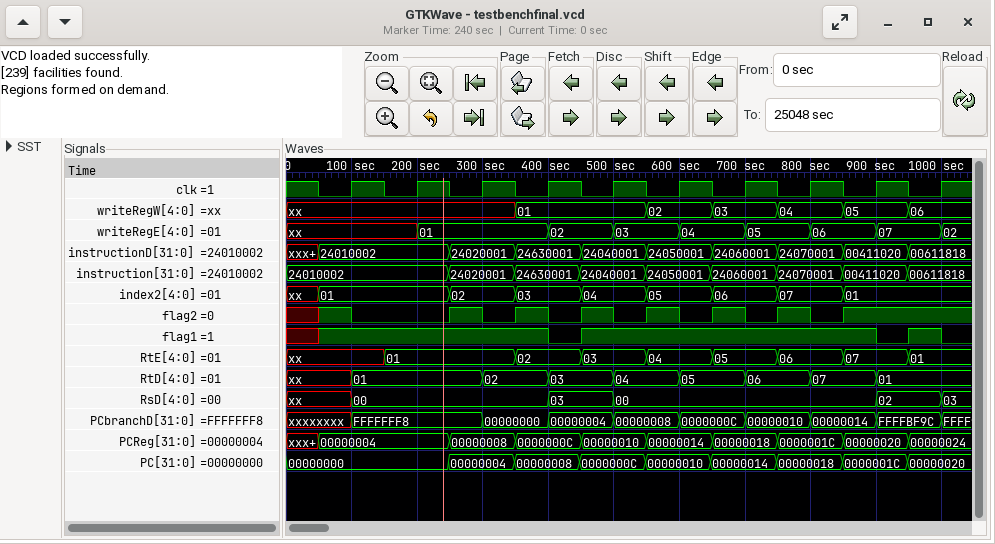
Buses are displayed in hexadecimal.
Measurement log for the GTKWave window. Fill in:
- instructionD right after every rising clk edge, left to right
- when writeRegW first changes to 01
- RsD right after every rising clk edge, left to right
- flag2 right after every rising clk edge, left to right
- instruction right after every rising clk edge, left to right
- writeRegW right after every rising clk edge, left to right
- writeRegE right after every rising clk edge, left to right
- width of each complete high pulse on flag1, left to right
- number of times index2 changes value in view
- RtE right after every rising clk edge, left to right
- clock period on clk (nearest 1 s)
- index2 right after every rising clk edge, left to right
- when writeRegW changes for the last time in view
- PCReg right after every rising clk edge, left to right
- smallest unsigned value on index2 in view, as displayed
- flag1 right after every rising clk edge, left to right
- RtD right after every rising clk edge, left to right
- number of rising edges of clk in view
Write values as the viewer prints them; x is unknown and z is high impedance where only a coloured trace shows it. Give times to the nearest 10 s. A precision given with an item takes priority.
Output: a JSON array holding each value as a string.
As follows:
["24010002, 24010002, 24020001, 24630001, 24040001, 24050001, 24060001, 24070001, 00411020, 00611818", "350 s", "00, 00, 00, 03, 00, 00, 00, 00, 02, 03", "0 0 0 0 0 0 0 0 1 1", "24010002, 24010002, 24020001, 24630001, 24040001, 24050001, 24060001, 24070001, 00411020, 00611818", "xx, xx, xx, 01, 01, 02, 03, 04, 05, 06", "xx, 01, 01, 02, 03, 04, 05, 06, 07, 02", "450 s, 50 s", "8", "xx, 01, 01, 02, 03, 04, 05, 06, 07, 01", "100 s", "01, 01, 02, 03, 04, 05, 06, 07, 01, 01", "950 s", "00000004, 00000004, 00000008, 0000000C, 00000010, 00000014, 00000018, 0000001C, 00000020, 00000024", "01", "1 1 1 0 1 1 1 1 0 0", "01, 01, 02, 03, 04, 05, 06, 07, 01, 01", "10"]
